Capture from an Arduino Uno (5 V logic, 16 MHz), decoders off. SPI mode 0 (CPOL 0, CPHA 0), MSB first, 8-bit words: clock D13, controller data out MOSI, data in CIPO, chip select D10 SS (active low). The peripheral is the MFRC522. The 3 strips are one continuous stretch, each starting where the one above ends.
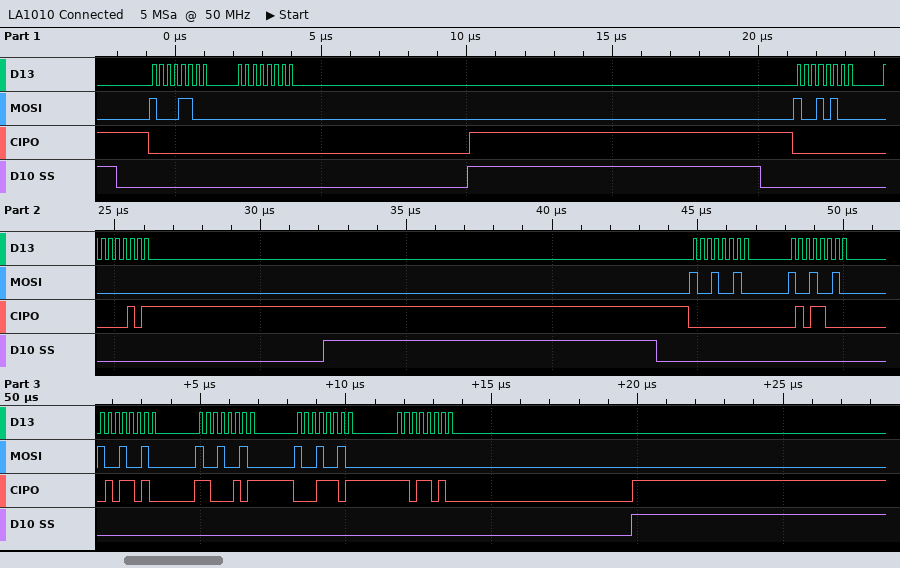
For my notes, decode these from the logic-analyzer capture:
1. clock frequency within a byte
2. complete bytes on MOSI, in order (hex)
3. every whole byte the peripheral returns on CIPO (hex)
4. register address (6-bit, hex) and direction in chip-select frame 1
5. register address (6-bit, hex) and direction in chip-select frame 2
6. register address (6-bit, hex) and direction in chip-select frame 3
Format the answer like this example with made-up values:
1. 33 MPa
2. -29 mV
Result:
1. 4 MHz
2. 8C 00 94 00 92 92 92 92 92 00
3. 00 00 00 05 00 58 5A C5 1D DA
4. 0x06 read
5. 0x0A read
6. 0x09 read
